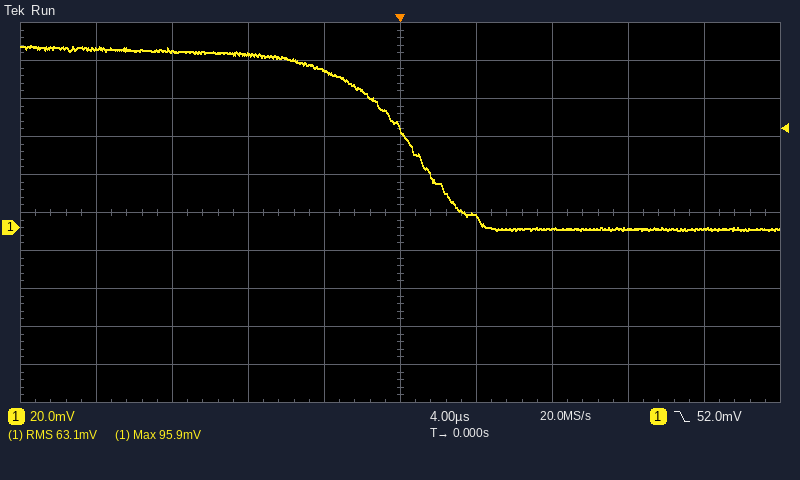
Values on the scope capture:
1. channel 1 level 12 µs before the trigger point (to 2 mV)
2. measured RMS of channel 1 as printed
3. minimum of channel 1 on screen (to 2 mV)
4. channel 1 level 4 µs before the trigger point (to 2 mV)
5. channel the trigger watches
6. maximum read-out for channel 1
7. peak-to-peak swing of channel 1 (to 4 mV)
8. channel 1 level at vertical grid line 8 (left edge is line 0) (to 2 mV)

94 mV
63.1 mV
-2 mV
82 mV
channel 1
95.9 mV
96 mV
0 mV
